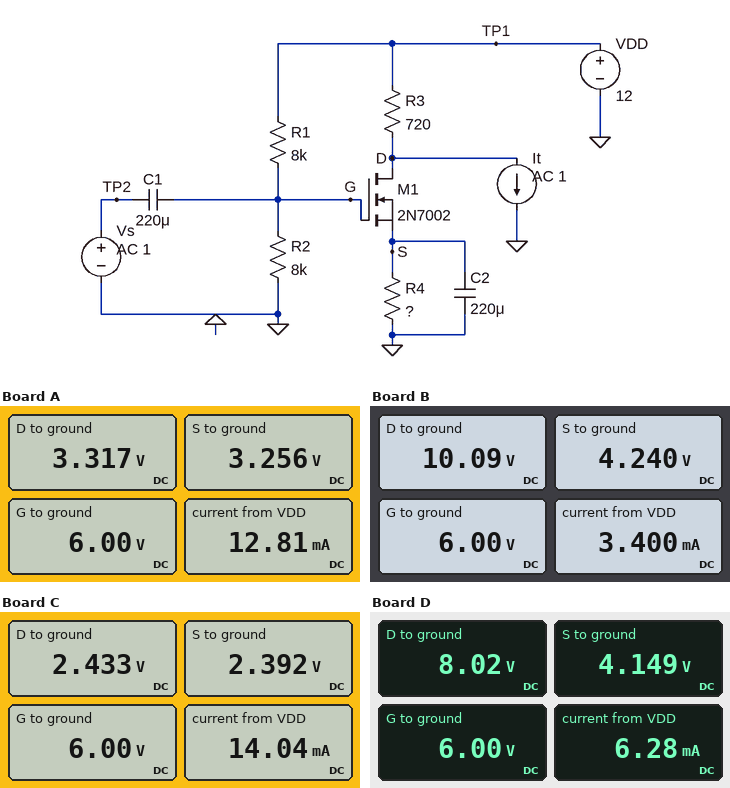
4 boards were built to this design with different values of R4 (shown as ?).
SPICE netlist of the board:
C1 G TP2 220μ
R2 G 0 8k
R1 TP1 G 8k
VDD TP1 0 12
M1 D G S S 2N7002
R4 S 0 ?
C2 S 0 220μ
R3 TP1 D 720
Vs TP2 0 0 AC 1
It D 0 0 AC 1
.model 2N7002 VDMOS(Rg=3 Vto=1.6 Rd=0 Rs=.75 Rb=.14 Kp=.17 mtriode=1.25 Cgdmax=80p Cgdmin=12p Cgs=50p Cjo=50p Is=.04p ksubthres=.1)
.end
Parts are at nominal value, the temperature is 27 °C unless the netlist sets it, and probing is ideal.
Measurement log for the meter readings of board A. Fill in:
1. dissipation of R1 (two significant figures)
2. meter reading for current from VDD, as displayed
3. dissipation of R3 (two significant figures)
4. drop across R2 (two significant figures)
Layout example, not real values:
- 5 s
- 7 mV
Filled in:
- 4.5 mW
- 12.81 mA
- 100 mW
- 6.0 V
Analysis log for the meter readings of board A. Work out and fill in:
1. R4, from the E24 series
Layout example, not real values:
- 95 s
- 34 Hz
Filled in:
- 270 Ω
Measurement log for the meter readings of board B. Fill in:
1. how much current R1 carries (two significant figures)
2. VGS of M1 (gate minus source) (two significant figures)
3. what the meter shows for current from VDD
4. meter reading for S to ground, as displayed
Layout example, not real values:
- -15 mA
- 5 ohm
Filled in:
- 750 µA
- 1.8 V
- 3.400 mA
- 4.240 V
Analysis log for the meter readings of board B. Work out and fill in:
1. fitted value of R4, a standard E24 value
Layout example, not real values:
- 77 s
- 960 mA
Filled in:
- 1.6 kΩ
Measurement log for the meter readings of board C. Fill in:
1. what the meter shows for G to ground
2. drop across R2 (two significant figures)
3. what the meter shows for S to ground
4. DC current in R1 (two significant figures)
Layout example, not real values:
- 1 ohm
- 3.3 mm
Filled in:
- 6.00 V
- 6.0 V
- 2.392 V
- 750 µA
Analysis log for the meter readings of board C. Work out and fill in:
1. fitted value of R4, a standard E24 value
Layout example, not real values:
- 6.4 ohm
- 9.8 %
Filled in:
- 180 Ω
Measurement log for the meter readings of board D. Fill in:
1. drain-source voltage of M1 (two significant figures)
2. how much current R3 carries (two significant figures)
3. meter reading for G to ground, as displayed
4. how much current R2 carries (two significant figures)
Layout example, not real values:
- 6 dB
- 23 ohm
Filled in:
- 3.9 V
- 5.5 mA
- 6.00 V
- 750 µA
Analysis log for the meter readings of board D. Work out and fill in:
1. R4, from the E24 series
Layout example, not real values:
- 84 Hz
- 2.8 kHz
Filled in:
- 750 Ω
